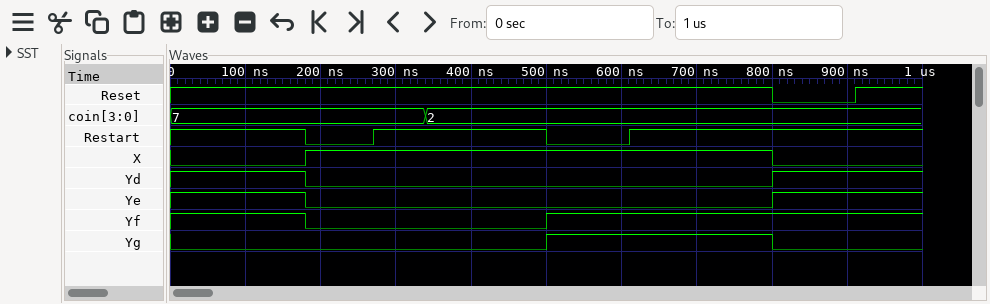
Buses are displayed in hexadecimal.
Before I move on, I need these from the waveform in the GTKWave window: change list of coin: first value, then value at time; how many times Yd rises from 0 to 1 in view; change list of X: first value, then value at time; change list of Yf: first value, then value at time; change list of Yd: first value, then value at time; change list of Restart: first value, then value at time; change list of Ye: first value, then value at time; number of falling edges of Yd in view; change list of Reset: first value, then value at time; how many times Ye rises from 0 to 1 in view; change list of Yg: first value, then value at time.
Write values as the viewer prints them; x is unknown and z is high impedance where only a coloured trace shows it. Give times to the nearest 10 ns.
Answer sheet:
7, 2 at 340 ns
1
0, 1 at 180 ns, 0 at 800 ns
1, 0 at 180 ns, 1 at 500 ns
1, 0 at 180 ns, 1 at 800 ns
1, 0 at 180 ns, 1 at 270 ns, 0 at 500 ns, 1 at 610 ns
1, 0 at 180 ns, 1 at 800 ns
1
1, 0 at 800 ns, 1 at 910 ns
1
0, 1 at 500 ns, 0 at 800 ns
